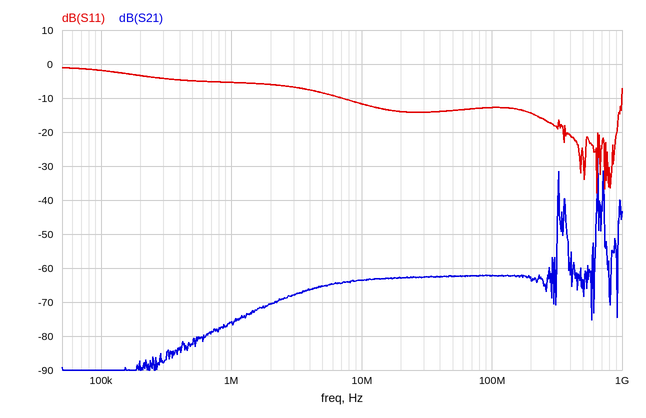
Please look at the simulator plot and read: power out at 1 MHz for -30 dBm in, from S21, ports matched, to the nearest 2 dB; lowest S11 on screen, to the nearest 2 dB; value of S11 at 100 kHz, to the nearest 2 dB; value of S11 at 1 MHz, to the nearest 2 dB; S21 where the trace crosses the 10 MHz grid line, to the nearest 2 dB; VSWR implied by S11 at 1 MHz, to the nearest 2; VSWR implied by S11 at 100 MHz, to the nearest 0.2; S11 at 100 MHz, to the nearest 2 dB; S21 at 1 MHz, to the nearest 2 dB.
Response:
-106 dBm
-38 dB
-2 dB
-6 dB
-64 dB
4
1.6
-12 dB
-76 dB
